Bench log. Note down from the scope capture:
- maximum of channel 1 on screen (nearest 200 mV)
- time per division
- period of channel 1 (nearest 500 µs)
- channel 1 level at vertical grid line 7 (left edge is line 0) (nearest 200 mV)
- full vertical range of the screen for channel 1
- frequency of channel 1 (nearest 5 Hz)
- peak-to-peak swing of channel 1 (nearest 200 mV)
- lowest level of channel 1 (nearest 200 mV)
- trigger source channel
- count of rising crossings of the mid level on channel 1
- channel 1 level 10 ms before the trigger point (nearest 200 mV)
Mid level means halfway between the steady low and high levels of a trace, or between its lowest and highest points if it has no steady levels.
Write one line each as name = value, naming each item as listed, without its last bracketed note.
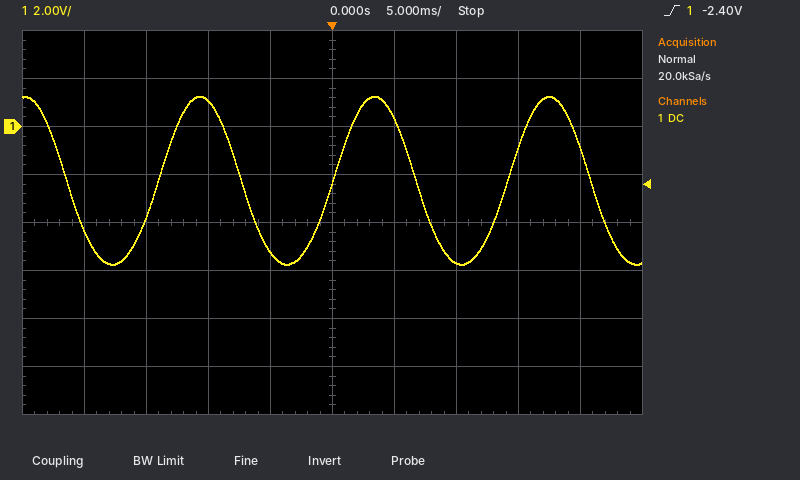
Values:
maximum of channel 1 on screen = 1.2 V
time per division = 5 ms
period of channel 1 = 14.0 ms
channel 1 level at vertical grid line 7 (left edge is line 0) = -5.6 V
full vertical range of the screen for channel 1 = 16 V
frequency of channel 1 = 70 Hz
peak-to-peak swing of channel 1 = 7.0 V
lowest level of channel 1 = -5.8 V
trigger source channel = channel 1
count of rising crossings of the mid level on channel 1 = 3
channel 1 level 10 ms before the trigger point = 1.0 V
